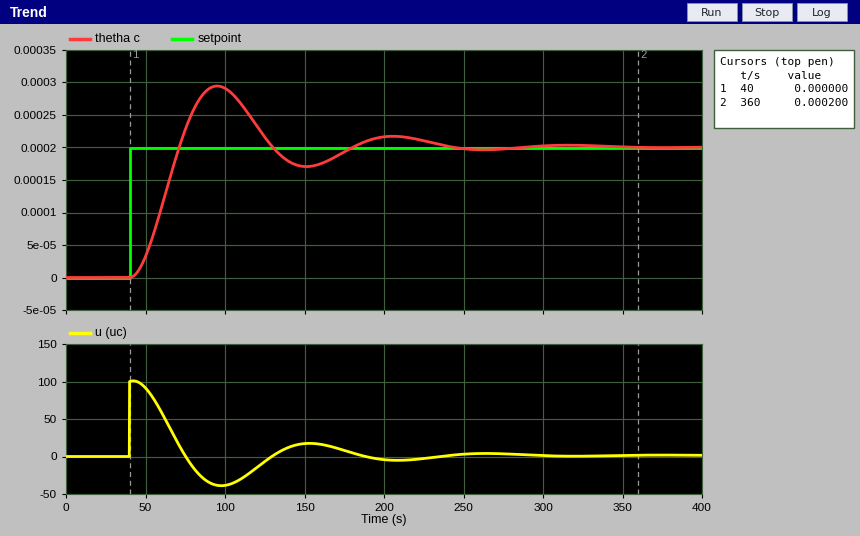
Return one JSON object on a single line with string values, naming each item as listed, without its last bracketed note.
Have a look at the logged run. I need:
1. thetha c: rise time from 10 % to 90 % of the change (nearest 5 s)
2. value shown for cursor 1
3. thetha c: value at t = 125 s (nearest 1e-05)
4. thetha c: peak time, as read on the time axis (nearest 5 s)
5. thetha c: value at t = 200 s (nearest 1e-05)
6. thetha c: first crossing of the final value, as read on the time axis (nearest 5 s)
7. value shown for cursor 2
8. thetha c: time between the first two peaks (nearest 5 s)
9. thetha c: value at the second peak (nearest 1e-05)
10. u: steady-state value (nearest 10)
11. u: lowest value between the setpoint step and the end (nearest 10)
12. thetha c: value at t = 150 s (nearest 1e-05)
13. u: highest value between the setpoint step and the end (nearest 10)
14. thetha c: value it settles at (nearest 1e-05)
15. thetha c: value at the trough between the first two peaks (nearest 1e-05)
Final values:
{"thetha c: rise time from 10 % to 90 % of the change": "20 s", "value shown for cursor 1": "0.000000", "thetha c: value at t = 125 s": "0.00022", "thetha c: peak time, as read on the time axis": "95 s", "thetha c: value at t = 200 s": "0.00022", "thetha c: first crossing of the final value, as read on the time axis": "70 s", "value shown for cursor 2": "0.000200", "thetha c: time between the first two peaks": "110 s", "thetha c: value at the second peak": "0.00022", "u: steady-state value": "0", "u: lowest value between the setpoint step and the end": "-40", "thetha c: value at t = 150 s": "0.00017", "u: highest value between the setpoint step and the end": "100", "thetha c: value it settles at": "0.00020", "thetha c: value at the trough between the first two peaks": "0.00017"}
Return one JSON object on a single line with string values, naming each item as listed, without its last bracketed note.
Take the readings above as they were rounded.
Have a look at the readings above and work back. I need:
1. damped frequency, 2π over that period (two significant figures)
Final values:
{"damped frequency, 2π over that period": "0.057 rad/s"}
